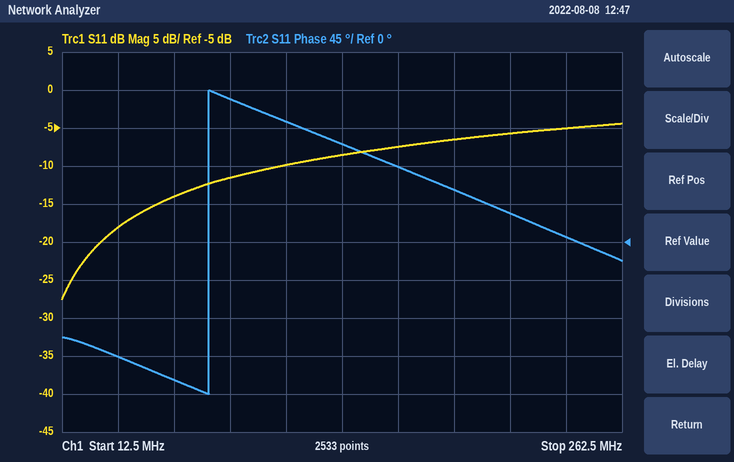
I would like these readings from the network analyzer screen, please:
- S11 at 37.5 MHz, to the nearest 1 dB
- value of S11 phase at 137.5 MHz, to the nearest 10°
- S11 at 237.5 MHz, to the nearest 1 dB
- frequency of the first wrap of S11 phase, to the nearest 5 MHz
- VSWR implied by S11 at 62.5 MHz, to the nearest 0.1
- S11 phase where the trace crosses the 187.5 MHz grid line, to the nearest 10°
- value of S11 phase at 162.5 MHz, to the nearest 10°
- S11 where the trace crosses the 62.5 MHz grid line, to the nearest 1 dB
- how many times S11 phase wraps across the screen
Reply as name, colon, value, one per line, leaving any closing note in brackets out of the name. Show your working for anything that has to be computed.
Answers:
S11 at 37.5 MHz, to the nearest 1 dB: -18 dB
value of S11 phase at 137.5 MHz, to the nearest 10°: 120°
S11 at 237.5 MHz, to the nearest 1 dB: -5 dB
frequency of the first wrap of S11 phase, to the nearest 5 MHz: 80 MHz
VSWR implied by S11 at 62.5 MHz, to the nearest 0.1: |Γ| = 10^(-14/20) = 0.1995; VSWR = (1 + 0.1995)/(1 − 0.1995) ≈ 1.5
S11 phase where the trace crosses the 187.5 MHz grid line, to the nearest 10°: 60°
value of S11 phase at 162.5 MHz, to the nearest 10°: 90°
S11 where the trace crosses the 62.5 MHz grid line, to the nearest 1 dB: -14 dB
how many times S11 phase wraps across the screen: 1
